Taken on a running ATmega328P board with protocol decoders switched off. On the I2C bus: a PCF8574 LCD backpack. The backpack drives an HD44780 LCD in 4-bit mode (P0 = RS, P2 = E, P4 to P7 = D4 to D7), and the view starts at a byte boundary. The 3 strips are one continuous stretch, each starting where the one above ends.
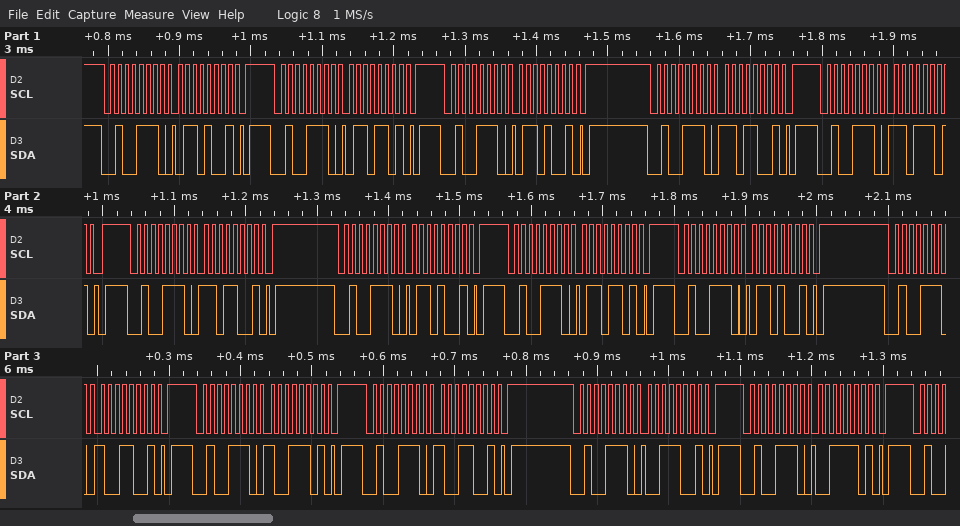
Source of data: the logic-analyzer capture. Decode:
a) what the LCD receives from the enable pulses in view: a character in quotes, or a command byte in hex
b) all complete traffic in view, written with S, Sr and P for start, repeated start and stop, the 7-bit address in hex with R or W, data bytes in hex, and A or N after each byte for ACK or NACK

'm' 'i'
S 27W A 69 A P S 27W A 6D A P S 27W A 69 A P S 27W A D9 A P S 27W A DD A P S 27W A D9 A P S 27W A 69 A P S 27W A 6D A P S 27W A 69 A P S 27W A 99 A P S 27W A 9D A P S 27W A 99 A P S 27W A 39 A P S 27W A 3D A P
